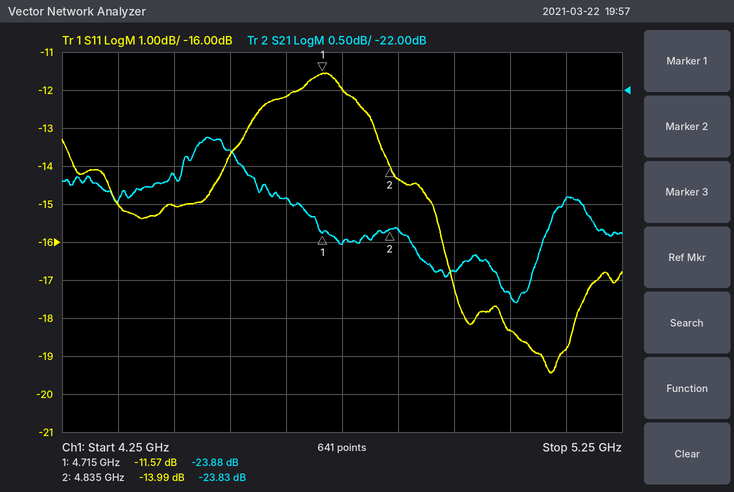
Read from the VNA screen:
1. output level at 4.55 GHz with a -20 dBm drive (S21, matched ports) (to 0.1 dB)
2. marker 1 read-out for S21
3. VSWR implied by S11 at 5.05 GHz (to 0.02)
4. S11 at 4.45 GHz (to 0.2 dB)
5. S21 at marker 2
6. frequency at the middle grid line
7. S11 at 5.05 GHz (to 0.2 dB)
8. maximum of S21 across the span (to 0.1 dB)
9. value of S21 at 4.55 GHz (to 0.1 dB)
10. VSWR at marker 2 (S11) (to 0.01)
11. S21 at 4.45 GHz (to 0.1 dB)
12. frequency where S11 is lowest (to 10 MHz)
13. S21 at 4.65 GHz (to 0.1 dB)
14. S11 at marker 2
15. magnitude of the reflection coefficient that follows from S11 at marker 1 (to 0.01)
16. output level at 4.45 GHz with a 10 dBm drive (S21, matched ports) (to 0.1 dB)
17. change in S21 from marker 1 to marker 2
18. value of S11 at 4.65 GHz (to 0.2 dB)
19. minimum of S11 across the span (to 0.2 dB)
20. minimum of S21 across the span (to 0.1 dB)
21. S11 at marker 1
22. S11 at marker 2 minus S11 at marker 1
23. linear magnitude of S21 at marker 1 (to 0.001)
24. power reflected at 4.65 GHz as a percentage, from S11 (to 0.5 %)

-42.8 dBm
-23.88 dB
1.28
-15.0 dB
-23.83 dB
4.75 GHz
-18.4 dB
-22.6 dB
-22.8 dB
1.50
-23.1 dB
5.12 GHz
-23.4 dB
-13.99 dB
0.26
-13.1 dBm
0.05 dB
-12.2 dB
-19.4 dB
-24.8 dB
-11.57 dB
-2.42 dB
0.064
6.0 %
